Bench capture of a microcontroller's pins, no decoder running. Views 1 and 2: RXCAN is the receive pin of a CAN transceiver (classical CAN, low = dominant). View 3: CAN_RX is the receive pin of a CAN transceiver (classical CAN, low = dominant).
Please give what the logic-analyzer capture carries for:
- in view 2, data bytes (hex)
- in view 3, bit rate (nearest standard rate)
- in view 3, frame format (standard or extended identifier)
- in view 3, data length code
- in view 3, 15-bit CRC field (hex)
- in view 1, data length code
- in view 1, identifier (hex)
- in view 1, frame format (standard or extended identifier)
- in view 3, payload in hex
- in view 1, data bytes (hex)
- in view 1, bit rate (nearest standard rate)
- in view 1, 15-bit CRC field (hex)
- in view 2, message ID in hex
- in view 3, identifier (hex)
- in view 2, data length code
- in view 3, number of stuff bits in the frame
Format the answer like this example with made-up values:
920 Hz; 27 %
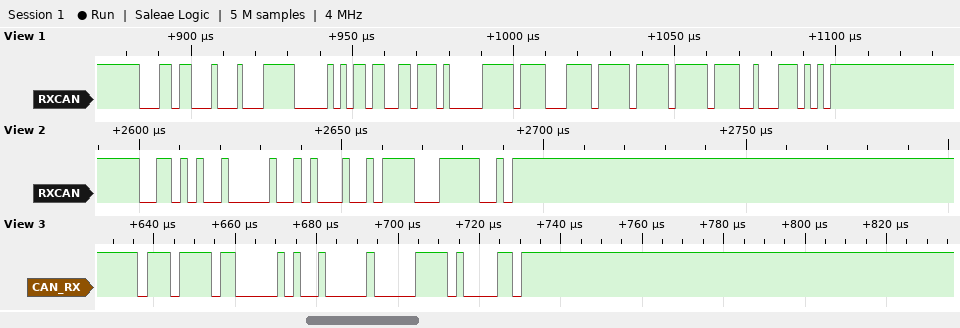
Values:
44; 500 kbit/s; standard; 1; 0x03A1; 8; 0x1B1; standard; 20; F8 2D 9B A0 FF 1E FF FF; 500 kbit/s; 0x723A; 0x352; 0x77B; 1; 3
